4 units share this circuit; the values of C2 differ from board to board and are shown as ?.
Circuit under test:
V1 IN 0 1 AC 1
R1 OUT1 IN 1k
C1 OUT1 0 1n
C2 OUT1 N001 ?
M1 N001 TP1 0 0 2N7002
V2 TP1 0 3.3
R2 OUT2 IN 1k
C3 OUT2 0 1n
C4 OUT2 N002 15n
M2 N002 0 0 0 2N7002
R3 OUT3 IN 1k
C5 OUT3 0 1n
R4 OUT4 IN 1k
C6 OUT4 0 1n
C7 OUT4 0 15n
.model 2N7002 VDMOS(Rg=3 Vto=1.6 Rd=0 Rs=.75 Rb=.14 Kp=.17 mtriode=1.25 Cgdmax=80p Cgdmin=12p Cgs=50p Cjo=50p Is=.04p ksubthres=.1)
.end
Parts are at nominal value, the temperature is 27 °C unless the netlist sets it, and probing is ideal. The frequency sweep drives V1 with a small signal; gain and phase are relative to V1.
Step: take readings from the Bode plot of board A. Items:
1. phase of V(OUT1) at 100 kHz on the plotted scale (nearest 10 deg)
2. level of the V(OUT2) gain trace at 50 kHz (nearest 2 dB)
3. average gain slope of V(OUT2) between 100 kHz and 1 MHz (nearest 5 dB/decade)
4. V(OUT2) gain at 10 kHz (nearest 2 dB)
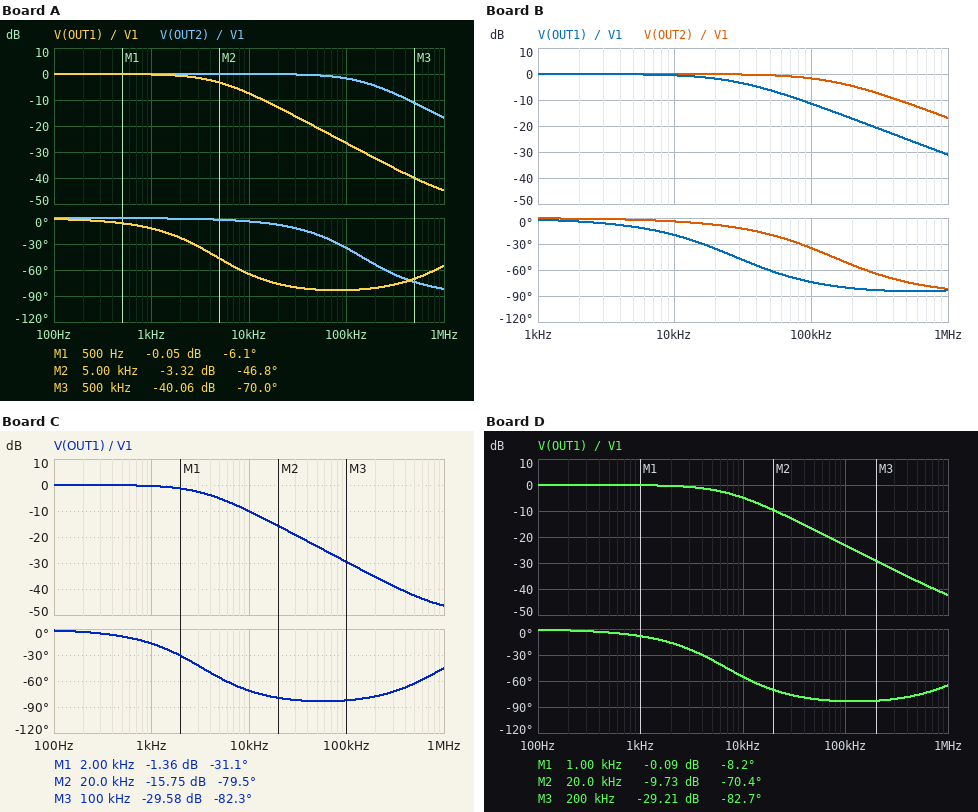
-80 deg
0 dB
-15 dB/decade
0 dB
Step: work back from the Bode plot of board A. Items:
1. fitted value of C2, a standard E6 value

33 nF
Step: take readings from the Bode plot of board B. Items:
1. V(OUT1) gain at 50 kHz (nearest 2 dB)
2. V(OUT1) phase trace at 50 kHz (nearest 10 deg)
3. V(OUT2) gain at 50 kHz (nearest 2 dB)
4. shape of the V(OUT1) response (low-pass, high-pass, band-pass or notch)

-6 dB
-60 deg
0 dB
low-pass
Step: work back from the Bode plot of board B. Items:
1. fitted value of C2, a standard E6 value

4.7 nF
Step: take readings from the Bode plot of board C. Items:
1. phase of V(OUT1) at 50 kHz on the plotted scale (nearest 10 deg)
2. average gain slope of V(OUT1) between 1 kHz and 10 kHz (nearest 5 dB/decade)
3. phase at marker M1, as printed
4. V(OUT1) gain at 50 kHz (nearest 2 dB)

-80 deg
-10 dB/decade
-31.1 deg
-24 dB
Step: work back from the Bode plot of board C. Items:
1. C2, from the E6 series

47 nF
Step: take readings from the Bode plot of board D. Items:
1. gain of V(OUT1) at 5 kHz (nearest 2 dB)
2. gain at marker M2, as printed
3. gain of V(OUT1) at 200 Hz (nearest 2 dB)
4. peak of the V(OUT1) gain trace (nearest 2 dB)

-2 dB
-9.73 dB
0 dB
0 dB
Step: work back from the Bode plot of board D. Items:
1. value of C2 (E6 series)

22 nF
